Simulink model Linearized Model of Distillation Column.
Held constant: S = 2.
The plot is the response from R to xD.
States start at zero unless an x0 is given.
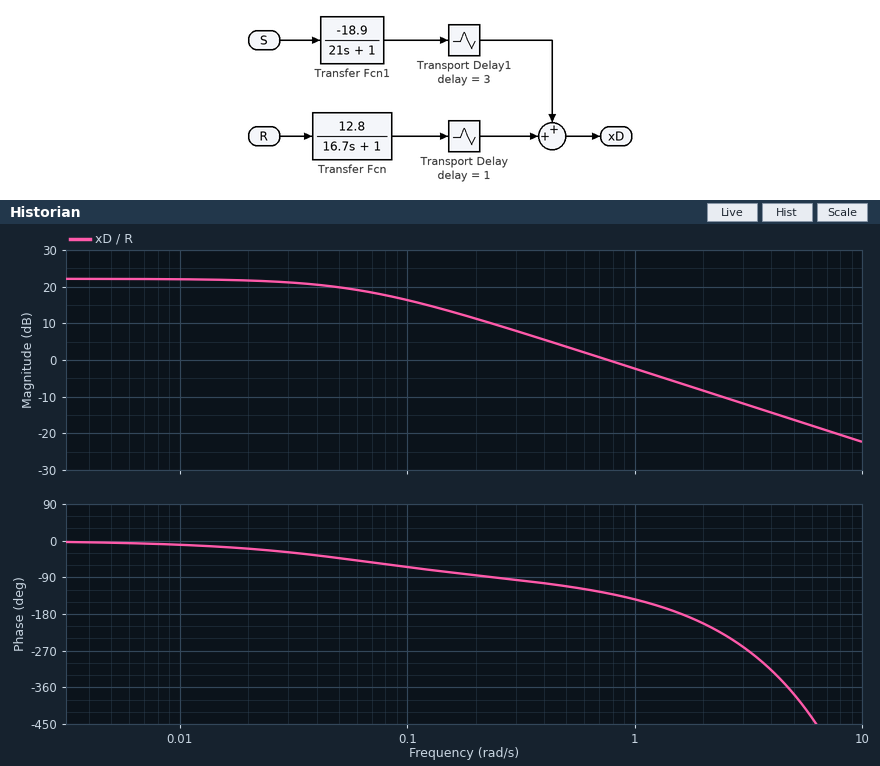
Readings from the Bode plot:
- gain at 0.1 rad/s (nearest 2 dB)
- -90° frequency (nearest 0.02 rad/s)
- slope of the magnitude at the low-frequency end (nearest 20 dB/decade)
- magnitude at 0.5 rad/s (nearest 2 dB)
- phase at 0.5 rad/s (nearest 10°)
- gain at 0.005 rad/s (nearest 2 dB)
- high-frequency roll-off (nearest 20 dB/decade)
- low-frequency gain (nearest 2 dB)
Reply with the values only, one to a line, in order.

16 dB
0.24 rad/s
0 dB/decade
4 dB
-110°
22 dB
-20 dB/decade
22 dB
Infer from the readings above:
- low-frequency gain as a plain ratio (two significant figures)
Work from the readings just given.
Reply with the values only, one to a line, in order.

13
